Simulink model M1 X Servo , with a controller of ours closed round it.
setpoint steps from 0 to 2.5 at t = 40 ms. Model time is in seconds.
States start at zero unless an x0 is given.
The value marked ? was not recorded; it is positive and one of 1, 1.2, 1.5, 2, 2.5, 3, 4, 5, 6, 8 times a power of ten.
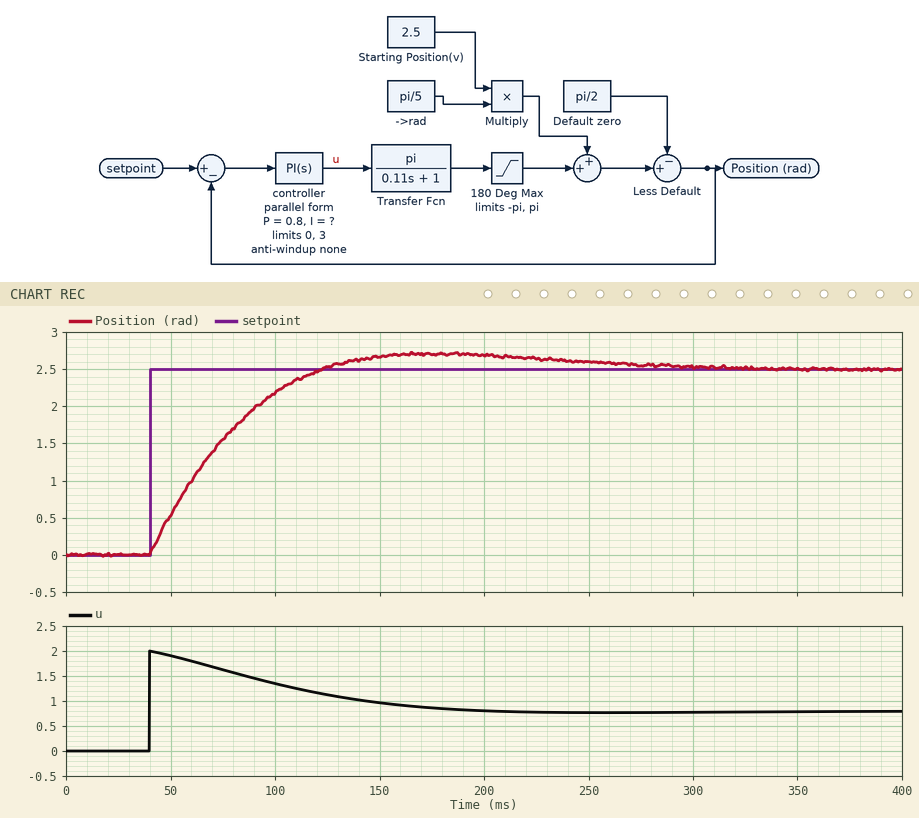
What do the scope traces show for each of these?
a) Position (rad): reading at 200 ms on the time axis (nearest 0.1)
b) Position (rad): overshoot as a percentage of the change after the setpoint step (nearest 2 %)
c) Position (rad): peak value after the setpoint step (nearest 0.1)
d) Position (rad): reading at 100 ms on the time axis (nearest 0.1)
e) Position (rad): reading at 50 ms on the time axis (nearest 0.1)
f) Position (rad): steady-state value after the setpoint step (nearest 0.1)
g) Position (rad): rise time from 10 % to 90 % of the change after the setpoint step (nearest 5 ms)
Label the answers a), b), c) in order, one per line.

a) 2.7
b) 8 %
c) 2.7
d) 2.2
e) 0.5
f) 2.5
g) 60 ms
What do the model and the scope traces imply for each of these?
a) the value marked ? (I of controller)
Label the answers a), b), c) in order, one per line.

a) 15
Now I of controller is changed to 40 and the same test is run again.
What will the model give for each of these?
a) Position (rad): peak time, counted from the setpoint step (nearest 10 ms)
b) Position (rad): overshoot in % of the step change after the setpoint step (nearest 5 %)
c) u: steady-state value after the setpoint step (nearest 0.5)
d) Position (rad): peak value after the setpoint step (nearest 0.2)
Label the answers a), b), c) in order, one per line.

a) 80 ms
b) 25 %
c) 1.0
d) 3.2
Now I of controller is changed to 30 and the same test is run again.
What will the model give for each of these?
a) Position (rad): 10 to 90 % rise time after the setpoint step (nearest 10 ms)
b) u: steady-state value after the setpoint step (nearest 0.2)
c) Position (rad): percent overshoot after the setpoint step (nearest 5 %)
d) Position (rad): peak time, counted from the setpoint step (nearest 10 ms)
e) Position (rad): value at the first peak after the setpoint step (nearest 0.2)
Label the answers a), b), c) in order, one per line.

a) 40 ms
b) 0.8
c) 20 %
d) 90 ms
e) 3.0
